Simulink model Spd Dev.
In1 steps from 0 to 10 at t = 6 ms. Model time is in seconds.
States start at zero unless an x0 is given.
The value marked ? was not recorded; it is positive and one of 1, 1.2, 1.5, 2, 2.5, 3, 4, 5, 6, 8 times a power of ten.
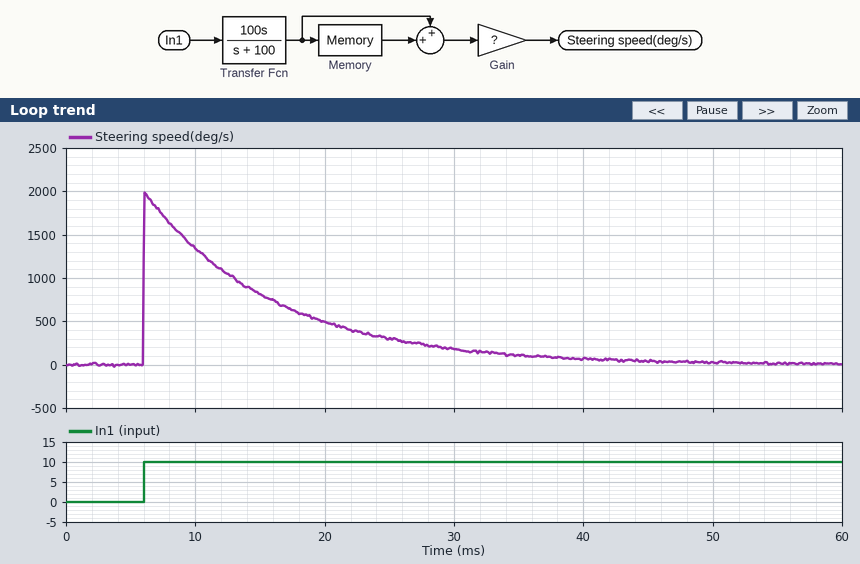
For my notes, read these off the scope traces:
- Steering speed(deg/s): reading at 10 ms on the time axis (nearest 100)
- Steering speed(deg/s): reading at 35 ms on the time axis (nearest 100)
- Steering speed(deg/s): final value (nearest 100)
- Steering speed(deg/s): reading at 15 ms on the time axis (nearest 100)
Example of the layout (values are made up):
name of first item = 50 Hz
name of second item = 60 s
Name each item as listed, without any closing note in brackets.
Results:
Steering speed(deg/s): reading at 10 ms on the time axis = 1300
Steering speed(deg/s): reading at 35 ms on the time axis = 100
Steering speed(deg/s): final value = 0
Steering speed(deg/s): reading at 15 ms on the time axis = 800
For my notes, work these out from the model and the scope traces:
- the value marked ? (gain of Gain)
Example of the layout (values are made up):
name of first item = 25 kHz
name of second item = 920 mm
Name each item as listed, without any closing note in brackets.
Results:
the value marked ? = 1
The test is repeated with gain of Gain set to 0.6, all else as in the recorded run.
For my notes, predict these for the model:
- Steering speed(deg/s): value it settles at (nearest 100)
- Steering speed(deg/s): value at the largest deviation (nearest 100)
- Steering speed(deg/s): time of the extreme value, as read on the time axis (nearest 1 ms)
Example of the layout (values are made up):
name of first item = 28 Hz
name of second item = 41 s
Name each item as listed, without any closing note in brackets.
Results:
Steering speed(deg/s): value it settles at = 0
Steering speed(deg/s): value at the largest deviation = 1200
Steering speed(deg/s): time of the extreme value, as read on the time axis = 6 ms
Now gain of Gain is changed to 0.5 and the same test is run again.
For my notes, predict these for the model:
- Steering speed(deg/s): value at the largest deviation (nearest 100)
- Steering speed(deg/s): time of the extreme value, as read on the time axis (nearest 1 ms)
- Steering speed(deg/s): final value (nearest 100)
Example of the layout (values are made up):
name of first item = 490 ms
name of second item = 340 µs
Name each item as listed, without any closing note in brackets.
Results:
Steering speed(deg/s): value at the largest deviation = 1000
Steering speed(deg/s): time of the extreme value, as read on the time axis = 6 ms
Steering speed(deg/s): final value = 0
